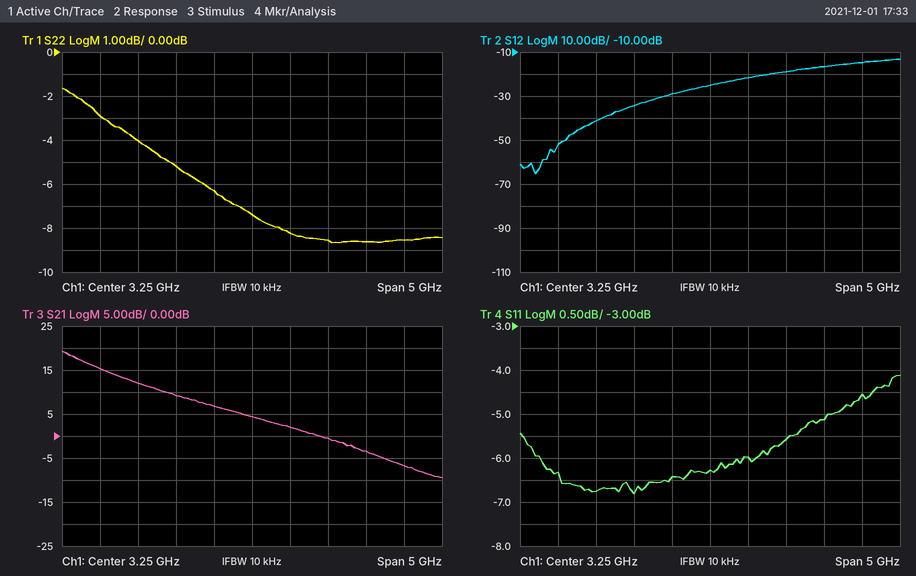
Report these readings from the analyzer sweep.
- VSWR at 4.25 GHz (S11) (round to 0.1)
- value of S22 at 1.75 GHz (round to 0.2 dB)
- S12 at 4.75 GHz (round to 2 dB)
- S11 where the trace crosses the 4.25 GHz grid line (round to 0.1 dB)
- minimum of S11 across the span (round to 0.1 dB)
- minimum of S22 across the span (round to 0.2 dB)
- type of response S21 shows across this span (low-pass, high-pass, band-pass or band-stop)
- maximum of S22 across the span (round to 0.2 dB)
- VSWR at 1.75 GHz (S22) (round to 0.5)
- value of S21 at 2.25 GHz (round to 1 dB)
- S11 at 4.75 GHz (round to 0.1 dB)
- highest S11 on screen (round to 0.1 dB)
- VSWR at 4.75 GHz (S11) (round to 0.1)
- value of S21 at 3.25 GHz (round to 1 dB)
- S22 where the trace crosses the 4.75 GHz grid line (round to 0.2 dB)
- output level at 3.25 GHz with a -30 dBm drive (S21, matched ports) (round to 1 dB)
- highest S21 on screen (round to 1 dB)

3.2
-4.0 dB
-16 dB
-5.6 dB
-6.8 dB
-8.6 dB
low-pass
-1.6 dB
4.5
9 dB
-5.1 dB
-4.1 dB
3.5
4 dB
-8.6 dB
-26 dBm
19 dB
